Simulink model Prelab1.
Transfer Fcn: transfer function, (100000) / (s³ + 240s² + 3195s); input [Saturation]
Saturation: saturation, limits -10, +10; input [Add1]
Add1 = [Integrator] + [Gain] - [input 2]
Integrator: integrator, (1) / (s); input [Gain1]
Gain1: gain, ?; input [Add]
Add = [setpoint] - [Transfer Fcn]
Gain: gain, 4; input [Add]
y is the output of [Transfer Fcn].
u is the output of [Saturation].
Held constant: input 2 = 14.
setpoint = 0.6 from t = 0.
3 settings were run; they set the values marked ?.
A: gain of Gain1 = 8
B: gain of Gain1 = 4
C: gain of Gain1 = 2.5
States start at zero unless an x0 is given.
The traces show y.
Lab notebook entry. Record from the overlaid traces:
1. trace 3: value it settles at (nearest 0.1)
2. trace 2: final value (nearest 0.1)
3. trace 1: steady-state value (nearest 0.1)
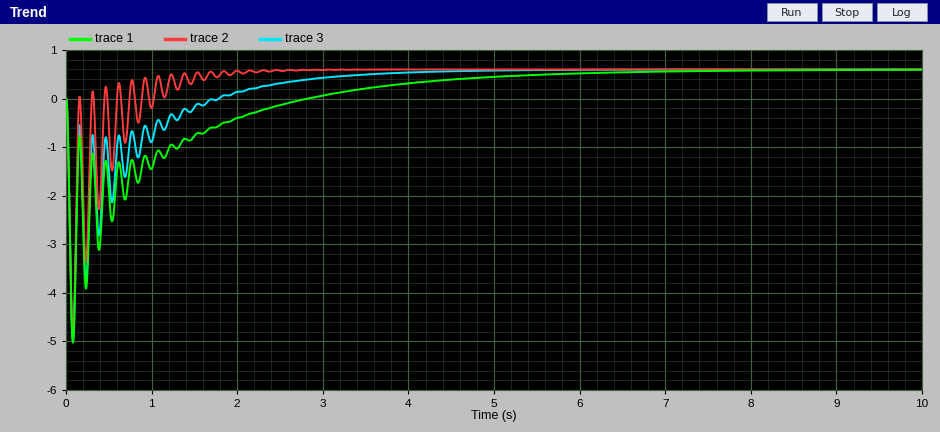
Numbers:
0.6
0.6
0.6
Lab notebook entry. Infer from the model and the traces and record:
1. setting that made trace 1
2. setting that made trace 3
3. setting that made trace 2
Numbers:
C
B
A
